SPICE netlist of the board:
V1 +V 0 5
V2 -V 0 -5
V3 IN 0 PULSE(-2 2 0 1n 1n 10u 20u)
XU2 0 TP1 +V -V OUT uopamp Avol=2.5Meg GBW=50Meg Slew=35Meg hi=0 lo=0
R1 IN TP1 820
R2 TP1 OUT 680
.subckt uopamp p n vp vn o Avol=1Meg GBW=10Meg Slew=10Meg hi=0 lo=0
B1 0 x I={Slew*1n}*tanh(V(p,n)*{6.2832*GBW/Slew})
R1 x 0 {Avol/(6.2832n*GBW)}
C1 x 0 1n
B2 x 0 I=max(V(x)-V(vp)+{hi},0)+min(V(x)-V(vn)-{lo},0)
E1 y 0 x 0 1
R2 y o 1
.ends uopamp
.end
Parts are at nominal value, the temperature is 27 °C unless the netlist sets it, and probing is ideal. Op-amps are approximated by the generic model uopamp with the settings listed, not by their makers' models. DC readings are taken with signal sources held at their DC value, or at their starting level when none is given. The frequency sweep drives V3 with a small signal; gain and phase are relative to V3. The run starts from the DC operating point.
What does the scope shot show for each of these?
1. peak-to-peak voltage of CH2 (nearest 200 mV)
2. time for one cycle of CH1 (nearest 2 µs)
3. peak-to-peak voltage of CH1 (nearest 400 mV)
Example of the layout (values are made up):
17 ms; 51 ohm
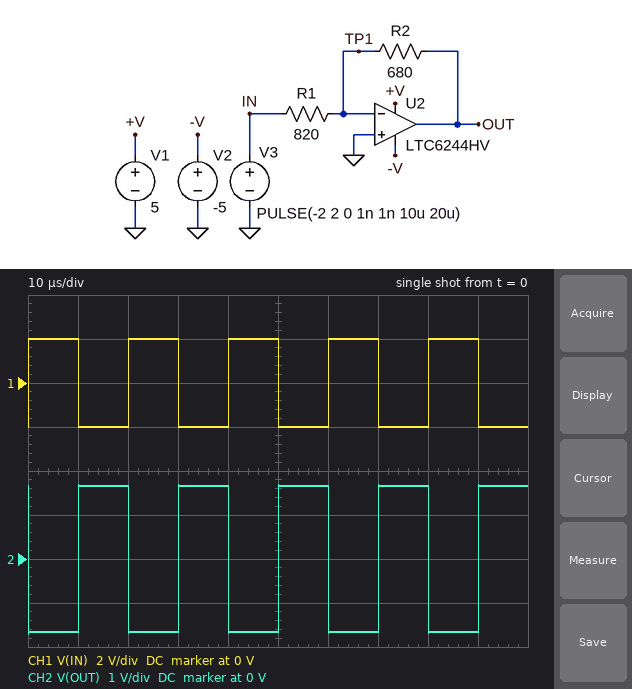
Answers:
3.4 V; 20 µs; 4.0 V
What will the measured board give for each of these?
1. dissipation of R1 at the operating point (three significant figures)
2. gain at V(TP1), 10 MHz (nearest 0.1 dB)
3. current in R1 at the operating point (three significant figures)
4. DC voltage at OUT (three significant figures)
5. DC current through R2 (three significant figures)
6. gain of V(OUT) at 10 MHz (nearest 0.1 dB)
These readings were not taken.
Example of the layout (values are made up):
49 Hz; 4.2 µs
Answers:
4.88 mW; -16.1 dB; 2.44 mA; 1.66 V; 2.44 mA; -2.2 dB
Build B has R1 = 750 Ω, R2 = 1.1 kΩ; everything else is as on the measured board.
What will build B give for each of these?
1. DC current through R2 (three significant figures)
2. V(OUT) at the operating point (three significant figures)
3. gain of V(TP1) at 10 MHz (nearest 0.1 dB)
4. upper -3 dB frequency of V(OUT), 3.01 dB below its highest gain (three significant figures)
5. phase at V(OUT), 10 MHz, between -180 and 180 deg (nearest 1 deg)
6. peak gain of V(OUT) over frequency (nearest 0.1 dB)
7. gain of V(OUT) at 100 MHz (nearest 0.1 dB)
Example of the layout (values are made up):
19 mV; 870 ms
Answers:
2.67 mA; 2.93 V; -11.6 dB; 20.3 MHz; 154 deg; 3.3 dB; -10.7 dB
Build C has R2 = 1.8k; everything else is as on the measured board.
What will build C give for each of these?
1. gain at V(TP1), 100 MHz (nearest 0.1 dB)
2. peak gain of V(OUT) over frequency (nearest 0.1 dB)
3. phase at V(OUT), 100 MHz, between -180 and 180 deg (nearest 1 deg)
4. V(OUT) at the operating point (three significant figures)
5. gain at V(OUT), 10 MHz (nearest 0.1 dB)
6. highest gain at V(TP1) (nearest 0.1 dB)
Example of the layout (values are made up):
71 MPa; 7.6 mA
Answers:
-3.4 dB; 6.8 dB; 99 deg; 4.39 V; 5.3 dB; -3.3 dB
